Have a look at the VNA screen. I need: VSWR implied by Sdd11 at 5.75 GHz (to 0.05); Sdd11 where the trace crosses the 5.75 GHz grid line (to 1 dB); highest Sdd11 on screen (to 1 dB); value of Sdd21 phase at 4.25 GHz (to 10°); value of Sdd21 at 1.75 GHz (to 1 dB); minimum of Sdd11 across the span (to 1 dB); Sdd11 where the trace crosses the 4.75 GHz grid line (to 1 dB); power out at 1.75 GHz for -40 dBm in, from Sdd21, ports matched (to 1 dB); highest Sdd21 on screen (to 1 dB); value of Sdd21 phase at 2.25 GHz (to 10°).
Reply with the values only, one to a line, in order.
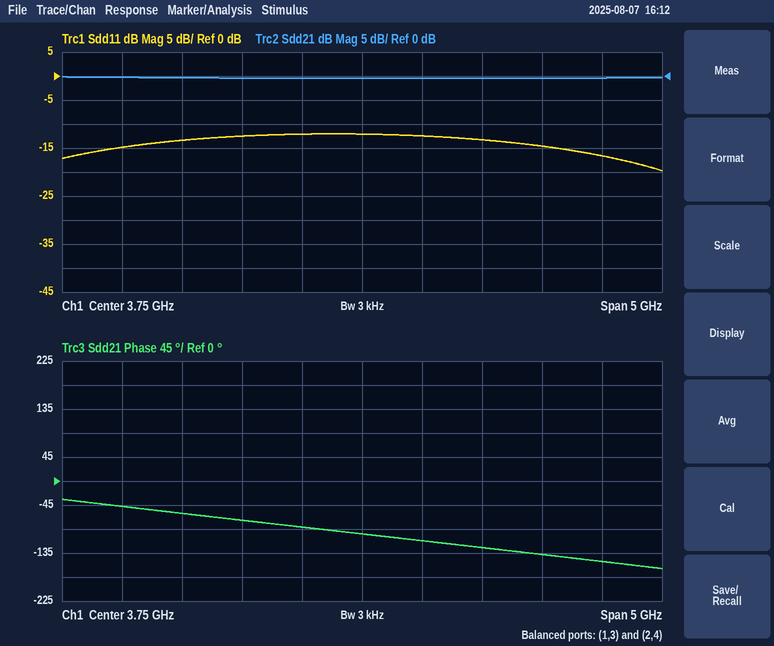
1.35
-17 dB
-12 dB
-110°
0 dB
-20 dB
-13 dB
-40 dBm
0 dB
-60°
